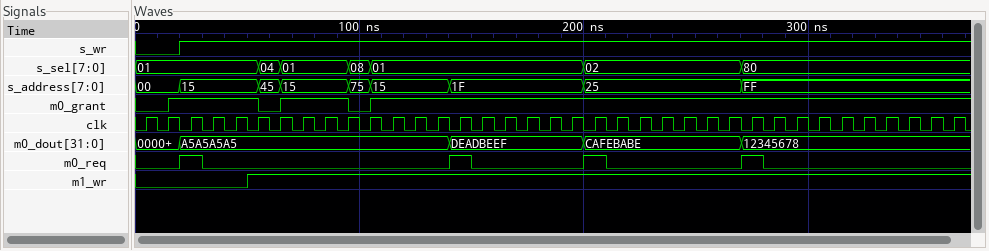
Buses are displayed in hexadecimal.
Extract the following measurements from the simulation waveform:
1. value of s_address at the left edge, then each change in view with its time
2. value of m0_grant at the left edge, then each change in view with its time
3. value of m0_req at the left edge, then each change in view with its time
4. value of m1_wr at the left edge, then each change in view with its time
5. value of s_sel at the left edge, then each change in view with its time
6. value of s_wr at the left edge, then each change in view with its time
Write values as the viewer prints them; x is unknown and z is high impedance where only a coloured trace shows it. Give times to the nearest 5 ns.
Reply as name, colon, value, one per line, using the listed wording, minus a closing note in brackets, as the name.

value of s_address at the left edge, then each change in view with its time: 00, 15 at 20 ns, 45 at 55 ns, 15 at 65 ns, 75 at 95 ns, 15 at 105 ns, 1F at 140 ns, 25 at 200 ns, FF at 270 ns
value of m0_grant at the left edge, then each change in view with its time: 0, 1 at 15 ns, 0 at 55 ns, 1 at 65 ns, 0 at 95 ns, 1 at 105 ns
value of m0_req at the left edge, then each change in view with its time: 0, 1 at 20 ns, 0 at 30 ns, 1 at 140 ns, 0 at 150 ns, 1 at 200 ns, 0 at 210 ns, 1 at 270 ns, 0 at 280 ns
value of m1_wr at the left edge, then each change in view with its time: 0, 1 at 50 ns
value of s_sel at the left edge, then each change in view with its time: 01, 04 at 55 ns, 01 at 65 ns, 08 at 95 ns, 01 at 105 ns, 02 at 200 ns, 80 at 270 ns
value of s_wr at the left edge, then each change in view with its time: 0, 1 at 20 ns
